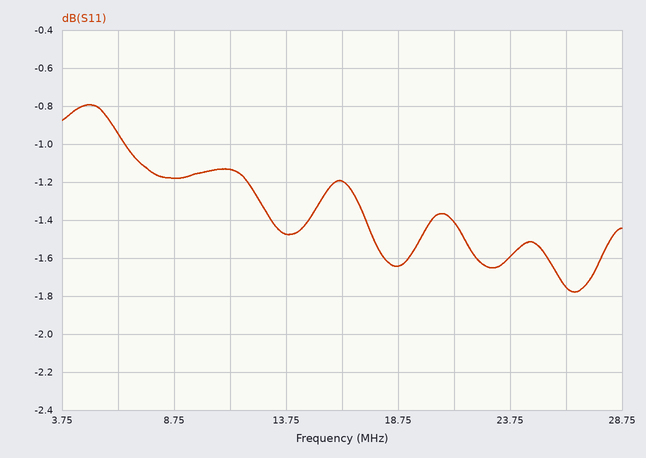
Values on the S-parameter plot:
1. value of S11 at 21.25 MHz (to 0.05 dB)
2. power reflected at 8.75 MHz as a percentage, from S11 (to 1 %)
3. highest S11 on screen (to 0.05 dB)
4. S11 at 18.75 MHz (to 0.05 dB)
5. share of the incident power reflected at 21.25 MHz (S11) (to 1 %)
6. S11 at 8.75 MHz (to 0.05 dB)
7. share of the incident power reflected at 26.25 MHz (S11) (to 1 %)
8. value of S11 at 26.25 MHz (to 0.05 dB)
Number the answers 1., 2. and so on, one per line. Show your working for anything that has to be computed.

1. -1.40 dB
2. 10^(-1.2/10) ≈ 76 %
3. -0.80 dB
4. -1.65 dB
5. 10^(-1.4/10) ≈ 72 %
6. -1.20 dB
7. 10^(-1.75/10) ≈ 67 %
8. -1.75 dB
